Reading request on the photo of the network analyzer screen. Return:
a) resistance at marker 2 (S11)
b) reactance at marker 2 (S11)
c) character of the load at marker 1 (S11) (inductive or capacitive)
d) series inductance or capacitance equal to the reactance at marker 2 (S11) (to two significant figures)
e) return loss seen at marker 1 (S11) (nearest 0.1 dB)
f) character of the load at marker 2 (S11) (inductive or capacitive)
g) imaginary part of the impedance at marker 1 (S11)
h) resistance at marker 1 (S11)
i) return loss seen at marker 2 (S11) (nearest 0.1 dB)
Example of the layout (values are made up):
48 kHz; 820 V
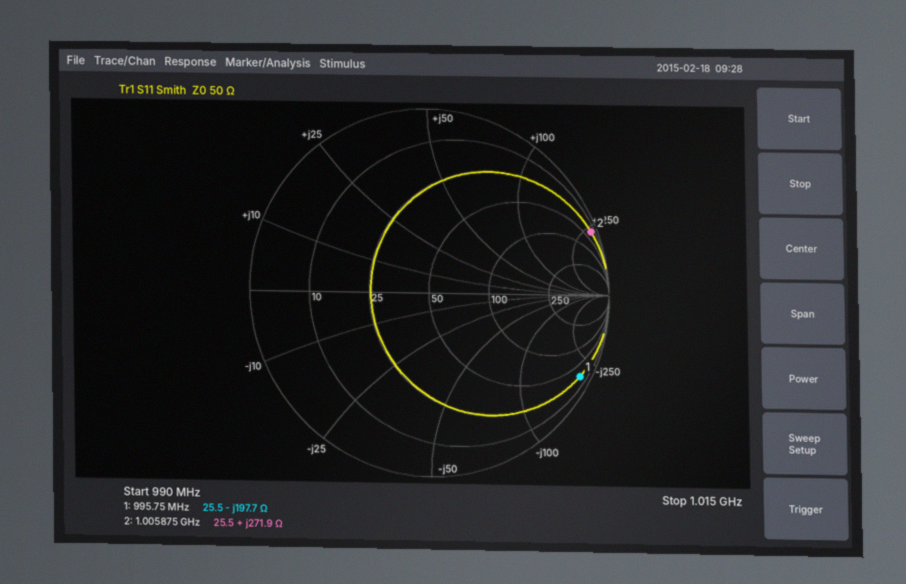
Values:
25.5 Ω; +271.9 Ω; capacitive; 43 nH; 0.5 dB; inductive; -197.7 Ω; 25.5 Ω; 0.3 dB
